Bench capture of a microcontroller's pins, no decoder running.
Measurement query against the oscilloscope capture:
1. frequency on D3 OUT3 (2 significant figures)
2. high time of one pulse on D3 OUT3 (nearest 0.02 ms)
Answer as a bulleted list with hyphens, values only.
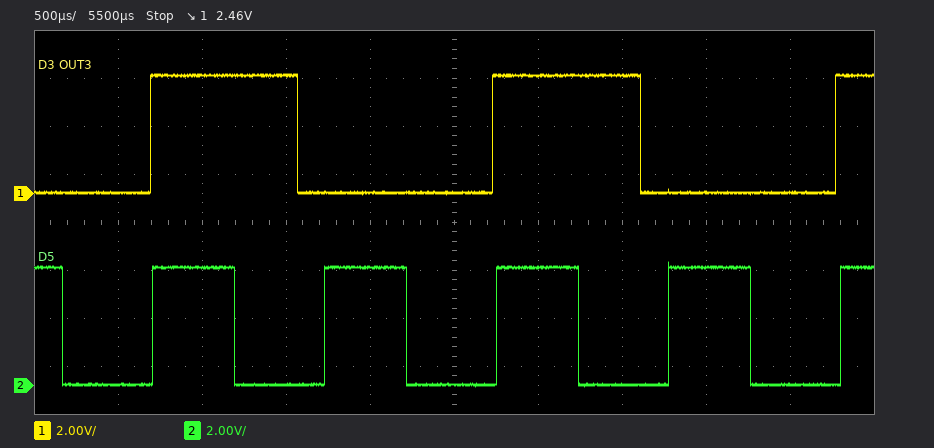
- 490 Hz
- 0.88 ms
